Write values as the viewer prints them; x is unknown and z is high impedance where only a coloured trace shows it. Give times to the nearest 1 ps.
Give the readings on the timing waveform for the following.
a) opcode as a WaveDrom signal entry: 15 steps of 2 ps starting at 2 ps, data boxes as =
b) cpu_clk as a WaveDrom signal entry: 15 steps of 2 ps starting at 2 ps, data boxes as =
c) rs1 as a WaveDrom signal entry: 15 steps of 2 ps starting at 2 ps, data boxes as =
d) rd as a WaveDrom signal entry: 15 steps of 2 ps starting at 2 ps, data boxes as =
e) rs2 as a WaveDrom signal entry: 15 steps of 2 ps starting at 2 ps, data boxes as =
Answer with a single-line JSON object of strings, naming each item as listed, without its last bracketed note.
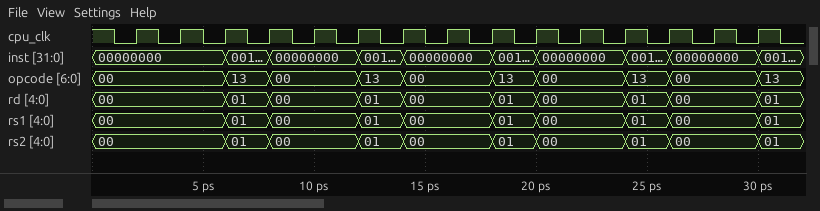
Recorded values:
{"opcode as a WaveDrom signal entry: 15 steps of 2 ps starting at 2 ps, data boxes as =": "{name: 'opcode', wave: '=.==.==.==.==.=', data: '00 13 00 13 00 13 00 13 00 13'}", "cpu_clk as a WaveDrom signal entry: 15 steps of 2 ps starting at 2 ps, data boxes as =": "{name: 'cpu_clk', wave: 'p..............'}", "rs1 as a WaveDrom signal entry: 15 steps of 2 ps starting at 2 ps, data boxes as =": "{name: 'rs1', wave: '=.==.==.==.==.=', data: '00 01 00 01 00 01 00 01 00 01'}", "rd as a WaveDrom signal entry: 15 steps of 2 ps starting at 2 ps, data boxes as =": "{name: 'rd', wave: '=.==.==.==.==.=', data: '00 01 00 01 00 01 00 01 00 01'}", "rs2 as a WaveDrom signal entry: 15 steps of 2 ps starting at 2 ps, data boxes as =": "{name: 'rs2', wave: '=.==.==.==.==.=', data: '00 01 00 01 00 01 00 01 00 01'}"}
